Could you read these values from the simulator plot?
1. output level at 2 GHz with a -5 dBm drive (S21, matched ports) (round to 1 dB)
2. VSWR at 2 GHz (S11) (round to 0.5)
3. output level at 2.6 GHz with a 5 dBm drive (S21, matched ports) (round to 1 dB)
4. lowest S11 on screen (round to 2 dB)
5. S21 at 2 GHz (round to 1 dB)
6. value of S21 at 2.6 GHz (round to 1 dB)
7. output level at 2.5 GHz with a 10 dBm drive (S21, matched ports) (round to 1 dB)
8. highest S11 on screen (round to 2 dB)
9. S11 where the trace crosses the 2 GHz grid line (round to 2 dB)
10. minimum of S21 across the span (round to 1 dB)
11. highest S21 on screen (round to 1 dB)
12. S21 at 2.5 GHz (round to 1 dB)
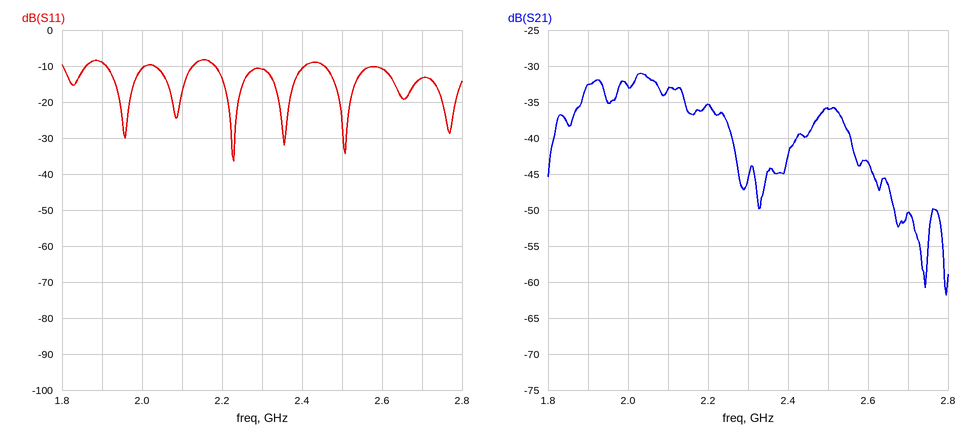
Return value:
-38 dBm
2.0
-38 dBm
-36 dB
-33 dB
-43 dB
-26 dBm
-8 dB
-10 dB
-62 dB
-31 dB
-36 dB
